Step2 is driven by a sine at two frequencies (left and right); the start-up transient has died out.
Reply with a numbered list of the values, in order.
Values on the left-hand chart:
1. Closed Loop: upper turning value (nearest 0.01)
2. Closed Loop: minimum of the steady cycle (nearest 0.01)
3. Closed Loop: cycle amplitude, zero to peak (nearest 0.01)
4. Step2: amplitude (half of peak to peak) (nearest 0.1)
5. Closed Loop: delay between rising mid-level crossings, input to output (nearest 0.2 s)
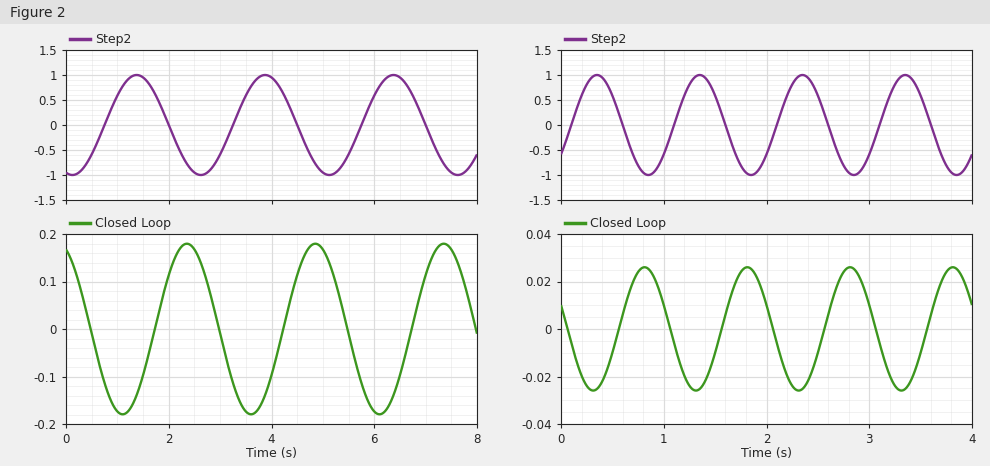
1. 0.18
2. -0.18
3. 0.18
4. 1.0
5. 1.0 s
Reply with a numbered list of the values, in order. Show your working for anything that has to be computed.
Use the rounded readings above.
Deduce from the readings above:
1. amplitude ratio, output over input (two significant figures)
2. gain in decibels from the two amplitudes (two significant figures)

1. 0.18 / 1 = 0.18
2. 20 log10(0.18 / 1) = -15 dB
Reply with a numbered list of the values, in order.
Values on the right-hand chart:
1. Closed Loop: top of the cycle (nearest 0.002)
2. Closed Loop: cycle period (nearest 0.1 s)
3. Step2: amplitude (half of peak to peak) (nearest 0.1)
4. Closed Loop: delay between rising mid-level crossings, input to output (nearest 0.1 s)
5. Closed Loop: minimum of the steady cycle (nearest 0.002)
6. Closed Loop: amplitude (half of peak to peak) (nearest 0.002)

1. 0.026
2. 1.0 s
3. 1.0
4. 0.5 s
5. -0.026
6. 0.026
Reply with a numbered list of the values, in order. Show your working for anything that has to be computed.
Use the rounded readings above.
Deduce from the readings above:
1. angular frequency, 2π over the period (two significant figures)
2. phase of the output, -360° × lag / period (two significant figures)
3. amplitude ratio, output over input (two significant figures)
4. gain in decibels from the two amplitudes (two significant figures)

1. 2π / 1 = 6.3 rad/s
2. -360 × 0.5 / 1 = -180°
3. 0.026 / 1 = 0.026
4. 20 log10(0.026 / 1) = -32 dB
